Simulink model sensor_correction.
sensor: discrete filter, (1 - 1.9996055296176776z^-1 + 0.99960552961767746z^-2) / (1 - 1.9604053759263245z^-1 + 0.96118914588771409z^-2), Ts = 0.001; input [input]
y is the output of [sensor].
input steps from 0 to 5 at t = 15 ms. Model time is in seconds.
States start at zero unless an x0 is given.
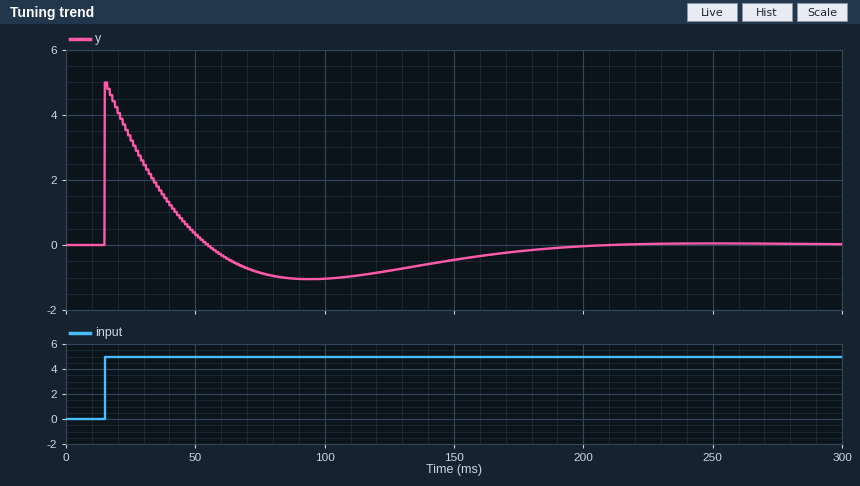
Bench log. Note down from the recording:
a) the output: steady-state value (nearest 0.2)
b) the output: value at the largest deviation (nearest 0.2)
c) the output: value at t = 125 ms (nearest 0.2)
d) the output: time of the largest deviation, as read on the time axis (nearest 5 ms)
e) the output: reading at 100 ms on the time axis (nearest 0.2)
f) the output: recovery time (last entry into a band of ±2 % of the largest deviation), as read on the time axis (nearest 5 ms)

0.0
5.0
-0.8
15 ms
-1.0
190 ms
